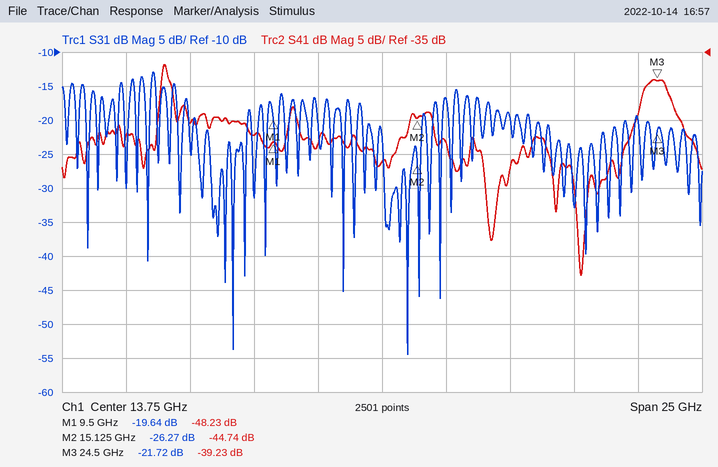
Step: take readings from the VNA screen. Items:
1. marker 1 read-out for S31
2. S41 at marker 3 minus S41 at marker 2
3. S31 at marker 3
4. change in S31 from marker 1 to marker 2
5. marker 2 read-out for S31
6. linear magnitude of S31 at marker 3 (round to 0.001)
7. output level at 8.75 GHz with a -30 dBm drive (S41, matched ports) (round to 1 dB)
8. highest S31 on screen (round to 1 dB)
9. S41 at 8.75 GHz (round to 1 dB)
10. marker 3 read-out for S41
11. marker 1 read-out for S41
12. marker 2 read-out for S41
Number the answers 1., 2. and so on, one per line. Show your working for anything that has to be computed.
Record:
1. -19.64 dB
2. -39.23 − (-44.74) = 5.51 dB
3. -21.72 dB
4. -26.27 − (-19.64) = -6.63 dB
5. -26.27 dB
6. 10^(-21.72/20) ≈ 0.082
7. -30 dBm + (-47 dB) = -77 dBm
8. -13 dB
9. -47 dB
10. -39.23 dB
11. -48.23 dB
12. -44.74 dB
